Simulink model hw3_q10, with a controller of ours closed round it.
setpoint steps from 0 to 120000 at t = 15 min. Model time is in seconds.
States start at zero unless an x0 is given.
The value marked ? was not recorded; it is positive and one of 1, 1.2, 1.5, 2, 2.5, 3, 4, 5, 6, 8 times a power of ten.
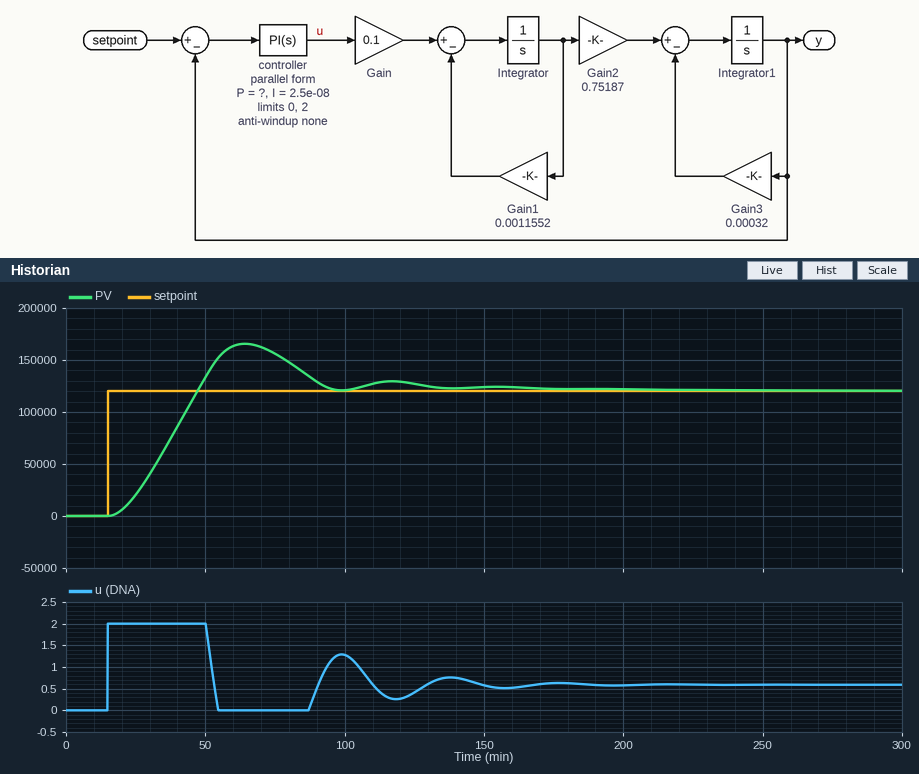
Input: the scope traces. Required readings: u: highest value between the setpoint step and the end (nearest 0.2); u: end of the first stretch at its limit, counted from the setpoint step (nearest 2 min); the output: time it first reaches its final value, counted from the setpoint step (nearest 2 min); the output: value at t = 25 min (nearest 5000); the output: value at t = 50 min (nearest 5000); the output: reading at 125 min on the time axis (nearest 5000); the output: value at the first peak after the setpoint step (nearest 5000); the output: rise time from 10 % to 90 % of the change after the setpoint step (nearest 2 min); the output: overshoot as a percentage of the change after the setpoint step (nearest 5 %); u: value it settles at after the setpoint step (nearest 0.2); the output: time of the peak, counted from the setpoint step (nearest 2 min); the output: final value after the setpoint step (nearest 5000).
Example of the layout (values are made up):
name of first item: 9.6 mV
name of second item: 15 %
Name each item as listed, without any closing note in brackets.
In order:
u: highest value between the setpoint step and the end: 2.0
u: end of the first stretch at its limit, counted from the setpoint step: 36 min
the output: time it first reaches its final value, counted from the setpoint step: 32 min
the output: value at t = 25 min: 20000
the output: value at t = 50 min: 135000
the output: reading at 125 min on the time axis: 125000
the output: value at the first peak after the setpoint step: 165000
the output: rise time from 10 % to 90 % of the change after the setpoint step: 22 min
the output: overshoot as a percentage of the change after the setpoint step: 40 %
u: value it settles at after the setpoint step: 0.6
the output: time of the peak, counted from the setpoint step: 50 min
the output: final value after the setpoint step: 120000
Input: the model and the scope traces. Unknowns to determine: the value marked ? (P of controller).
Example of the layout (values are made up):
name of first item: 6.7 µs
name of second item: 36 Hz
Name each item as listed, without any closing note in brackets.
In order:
the value marked ?: 0.0001
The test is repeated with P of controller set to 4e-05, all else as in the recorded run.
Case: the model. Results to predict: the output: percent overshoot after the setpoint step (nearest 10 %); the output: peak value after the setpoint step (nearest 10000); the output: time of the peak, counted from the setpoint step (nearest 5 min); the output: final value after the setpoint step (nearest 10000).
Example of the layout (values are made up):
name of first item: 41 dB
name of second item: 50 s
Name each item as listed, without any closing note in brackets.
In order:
the output: percent overshoot after the setpoint step: 60 %
the output: peak value after the setpoint step: 190000
the output: time of the peak, counted from the setpoint step: 55 min
the output: final value after the setpoint step: 120000
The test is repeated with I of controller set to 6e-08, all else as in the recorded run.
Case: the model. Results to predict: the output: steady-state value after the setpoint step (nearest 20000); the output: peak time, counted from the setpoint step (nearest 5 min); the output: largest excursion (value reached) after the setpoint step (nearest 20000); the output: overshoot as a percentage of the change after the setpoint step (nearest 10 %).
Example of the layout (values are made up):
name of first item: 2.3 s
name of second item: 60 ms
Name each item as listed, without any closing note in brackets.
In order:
the output: steady-state value after the setpoint step: 120000
the output: peak time, counted from the setpoint step: 55 min
the output: largest excursion (value reached) after the setpoint step: 200000
the output: overshoot as a percentage of the change after the setpoint step: 60 %
